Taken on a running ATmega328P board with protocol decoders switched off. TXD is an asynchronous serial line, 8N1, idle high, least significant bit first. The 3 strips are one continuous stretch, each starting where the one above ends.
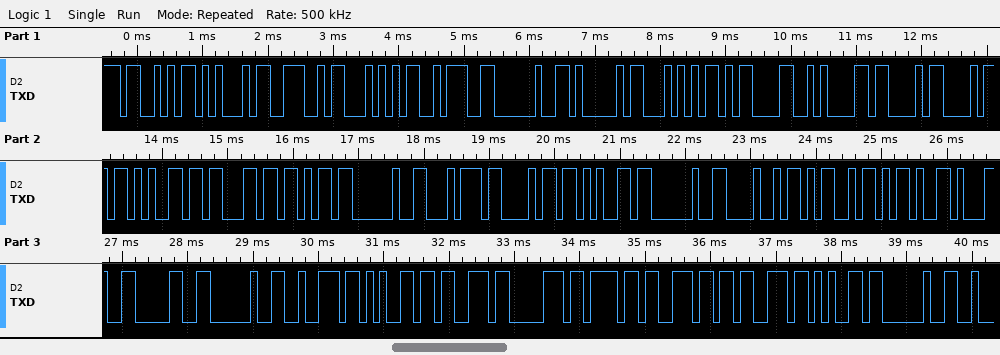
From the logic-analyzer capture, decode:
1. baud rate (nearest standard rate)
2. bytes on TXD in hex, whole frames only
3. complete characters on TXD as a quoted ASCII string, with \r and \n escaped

9600 baud
0x53 0x45 0x4E 0x54 0x3A 0x20 0x41 0x54 0x0D 0x0A 0x43 0x68 0x65 0x63 0x6B 0x20 0x74 0x68 0x65 0x20 0x48 0x4D 0x2D 0x31 0x30 0x20 0x72 0x65 0x73 0x70 0x6F 0x6E 0x73 0x65 0x20
"SENT: AT\r\nCheck the HM-10 response "
